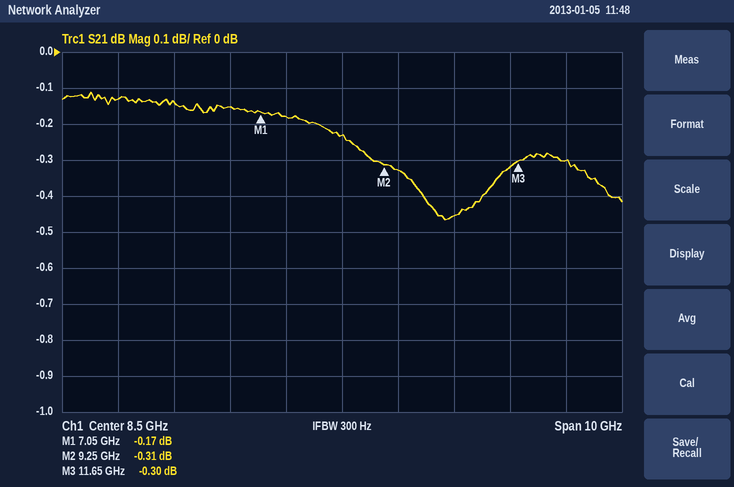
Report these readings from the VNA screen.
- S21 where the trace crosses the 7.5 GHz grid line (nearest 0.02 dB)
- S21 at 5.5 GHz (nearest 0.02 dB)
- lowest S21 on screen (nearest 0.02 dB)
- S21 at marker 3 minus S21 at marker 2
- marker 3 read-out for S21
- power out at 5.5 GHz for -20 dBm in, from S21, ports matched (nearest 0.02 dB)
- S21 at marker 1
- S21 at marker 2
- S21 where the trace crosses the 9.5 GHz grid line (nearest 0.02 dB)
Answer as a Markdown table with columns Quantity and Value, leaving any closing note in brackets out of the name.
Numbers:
| Quantity | Value |
|---|---|
| S21 where the trace crosses the 7.5 GHz grid line | -0.18 dB |
| S21 at 5.5 GHz | -0.14 dB |
| lowest S21 on screen | -0.46 dB |
| S21 at marker 3 minus S21 at marker 2 | 0.01 dB |
| marker 3 read-out for S21 | -0.30 dB |
| power out at 5.5 GHz for -20 dBm in, from S21, ports matched | -20.14 dBm |
| S21 at marker 1 | -0.17 dB |
| S21 at marker 2 | -0.31 dB |
| S21 where the trace crosses the 9.5 GHz grid line | -0.32 dB |
